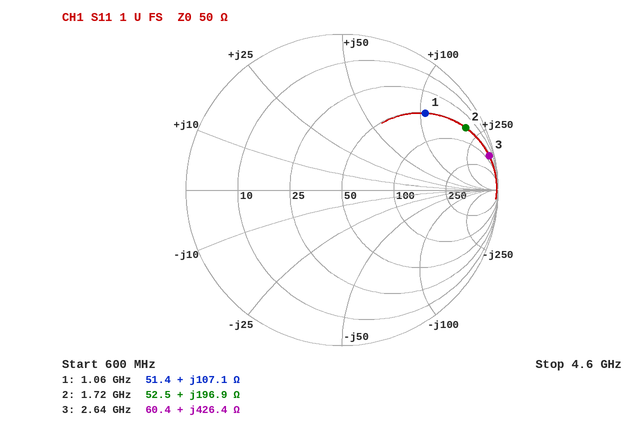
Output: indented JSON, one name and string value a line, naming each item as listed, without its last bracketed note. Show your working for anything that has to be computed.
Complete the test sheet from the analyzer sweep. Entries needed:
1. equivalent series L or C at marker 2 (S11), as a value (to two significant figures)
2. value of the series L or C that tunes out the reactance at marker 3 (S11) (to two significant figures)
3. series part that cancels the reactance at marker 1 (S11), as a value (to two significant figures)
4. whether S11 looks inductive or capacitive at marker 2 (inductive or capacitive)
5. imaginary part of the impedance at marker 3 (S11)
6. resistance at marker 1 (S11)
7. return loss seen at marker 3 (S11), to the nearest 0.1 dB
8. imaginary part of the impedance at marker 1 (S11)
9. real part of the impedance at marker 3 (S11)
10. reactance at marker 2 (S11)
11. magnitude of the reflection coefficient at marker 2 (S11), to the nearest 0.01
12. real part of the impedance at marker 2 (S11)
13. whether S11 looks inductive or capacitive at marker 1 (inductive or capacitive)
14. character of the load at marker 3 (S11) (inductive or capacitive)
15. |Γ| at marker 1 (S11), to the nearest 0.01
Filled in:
{
  "equivalent series L or C at marker 2 (S11), as a value": "L = 196.9 Ω/(2π × 1.72 GHz) ≈ 18 nH",
  "value of the series L or C that tunes out the reactance at marker 3 (S11)": "C = 1/(2π × 2.64 GHz × 426.4 Ω) ≈ 141 fF, so 140 fF to two significant figures",
  "series part that cancels the reactance at marker 1 (S11), as a value": "C = 1/(2π × 1.06 GHz × 107.1 Ω) ≈ 1.4 pF",
  "whether S11 looks inductive or capacitive at marker 2": "inductive",
  "imaginary part of the impedance at marker 3": "+426.4 Ω",
  "resistance at marker 1": "51.4 Ω",
  "return loss seen at marker 3 (S11), to the nearest 0.1 dB": "0.3 dB",
  "imaginary part of the impedance at marker 1": "+107.1 Ω",
  "real part of the impedance at marker 3": "60.4 Ω",
  "reactance at marker 2": "+196.9 Ω",
  "magnitude of the reflection coefficient at marker 2 (S11), to the nearest 0.01": "0.89",
  "real part of the impedance at marker 2": "52.5 Ω",
  "whether S11 looks inductive or capacitive at marker 1": "inductive",
  "character of the load at marker 3 (S11)": "inductive",
  "|Γ| at marker 1 (S11), to the nearest 0.01": "0.73"
}
